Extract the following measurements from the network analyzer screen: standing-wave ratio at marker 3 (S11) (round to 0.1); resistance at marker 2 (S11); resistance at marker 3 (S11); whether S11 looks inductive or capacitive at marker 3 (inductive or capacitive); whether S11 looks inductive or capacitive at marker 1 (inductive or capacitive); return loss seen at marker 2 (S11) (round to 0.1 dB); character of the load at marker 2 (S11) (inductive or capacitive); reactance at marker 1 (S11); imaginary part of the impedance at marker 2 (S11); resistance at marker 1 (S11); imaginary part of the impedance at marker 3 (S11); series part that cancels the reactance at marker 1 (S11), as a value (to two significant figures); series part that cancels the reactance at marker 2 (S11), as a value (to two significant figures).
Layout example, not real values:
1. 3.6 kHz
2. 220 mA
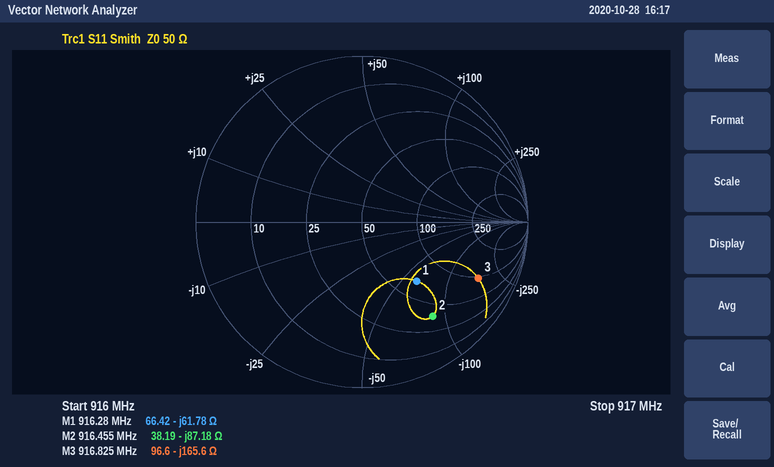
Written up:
1. 8.0
2. 38.19 Ω
3. 96.6 Ω
4. capacitive
5. capacitive
6. 3.0 dB
7. capacitive
8. -61.78 Ω
9. -87.18 Ω
10. 66.42 Ω
11. -165.6 Ω
12. 11 nH
13. 15 nH
